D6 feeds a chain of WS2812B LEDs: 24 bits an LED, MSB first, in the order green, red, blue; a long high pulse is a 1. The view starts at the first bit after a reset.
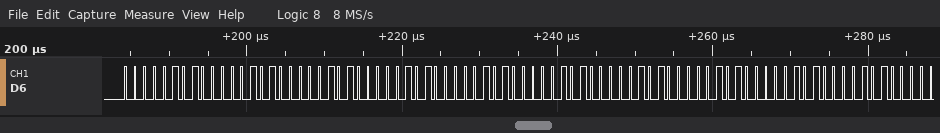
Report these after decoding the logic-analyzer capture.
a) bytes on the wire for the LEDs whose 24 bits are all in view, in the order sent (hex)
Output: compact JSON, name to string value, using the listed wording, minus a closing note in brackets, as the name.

{"bytes on the wire for the LEDs whose 24 bits are all in view, in the order sent": "05 05 05 05 05 05 05 05 05"}
